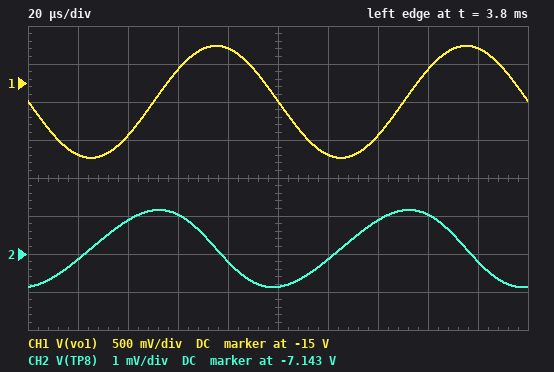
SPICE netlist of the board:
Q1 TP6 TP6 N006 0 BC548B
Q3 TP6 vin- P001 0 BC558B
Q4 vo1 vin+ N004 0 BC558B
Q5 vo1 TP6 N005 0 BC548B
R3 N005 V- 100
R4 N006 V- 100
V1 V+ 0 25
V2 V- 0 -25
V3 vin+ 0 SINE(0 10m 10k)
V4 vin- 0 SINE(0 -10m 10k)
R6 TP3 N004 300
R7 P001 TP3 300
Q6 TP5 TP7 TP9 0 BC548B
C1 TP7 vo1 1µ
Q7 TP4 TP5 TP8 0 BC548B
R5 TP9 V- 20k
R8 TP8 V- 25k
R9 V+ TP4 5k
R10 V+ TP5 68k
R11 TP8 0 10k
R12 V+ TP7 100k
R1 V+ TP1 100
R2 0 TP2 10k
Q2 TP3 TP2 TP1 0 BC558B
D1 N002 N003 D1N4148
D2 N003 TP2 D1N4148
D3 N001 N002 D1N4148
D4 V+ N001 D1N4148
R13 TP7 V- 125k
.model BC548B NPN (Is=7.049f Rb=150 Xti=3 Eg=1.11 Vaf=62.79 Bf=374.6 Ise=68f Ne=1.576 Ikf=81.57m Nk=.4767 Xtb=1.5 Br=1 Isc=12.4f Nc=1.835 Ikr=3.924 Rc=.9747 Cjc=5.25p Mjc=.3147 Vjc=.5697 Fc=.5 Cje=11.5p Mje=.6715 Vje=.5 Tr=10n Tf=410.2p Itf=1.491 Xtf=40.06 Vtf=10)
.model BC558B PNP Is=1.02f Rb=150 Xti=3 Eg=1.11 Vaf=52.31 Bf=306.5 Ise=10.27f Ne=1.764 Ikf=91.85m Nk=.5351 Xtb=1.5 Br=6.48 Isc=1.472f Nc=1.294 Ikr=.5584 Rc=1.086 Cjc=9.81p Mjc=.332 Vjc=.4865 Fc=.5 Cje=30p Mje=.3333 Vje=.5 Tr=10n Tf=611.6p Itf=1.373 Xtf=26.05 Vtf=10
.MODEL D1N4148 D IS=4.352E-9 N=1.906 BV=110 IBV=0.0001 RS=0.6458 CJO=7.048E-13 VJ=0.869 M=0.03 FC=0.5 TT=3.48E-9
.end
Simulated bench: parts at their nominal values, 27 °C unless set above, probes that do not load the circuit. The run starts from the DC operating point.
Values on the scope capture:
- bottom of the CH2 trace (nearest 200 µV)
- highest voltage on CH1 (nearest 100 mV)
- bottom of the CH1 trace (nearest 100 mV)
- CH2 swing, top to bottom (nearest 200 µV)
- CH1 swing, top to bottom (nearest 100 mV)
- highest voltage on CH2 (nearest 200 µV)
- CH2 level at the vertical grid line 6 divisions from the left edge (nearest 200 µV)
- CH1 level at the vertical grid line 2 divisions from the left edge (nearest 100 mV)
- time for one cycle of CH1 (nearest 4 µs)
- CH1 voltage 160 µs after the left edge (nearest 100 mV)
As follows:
-7.1438 V
-14.5 V
-16.0 V
2.0 mV
1.5 V
-7.1418 V
-7.1432 V
-15.7 V
100 µs
-14.8 V
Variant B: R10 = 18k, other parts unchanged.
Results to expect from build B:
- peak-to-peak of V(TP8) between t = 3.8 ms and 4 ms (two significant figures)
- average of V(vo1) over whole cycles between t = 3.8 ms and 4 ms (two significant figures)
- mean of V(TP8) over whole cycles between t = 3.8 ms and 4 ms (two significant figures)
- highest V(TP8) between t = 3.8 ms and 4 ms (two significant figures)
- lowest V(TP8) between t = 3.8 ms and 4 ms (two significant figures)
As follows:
1.9 V
-16 V
1.5 V
2.6 V
760 mV
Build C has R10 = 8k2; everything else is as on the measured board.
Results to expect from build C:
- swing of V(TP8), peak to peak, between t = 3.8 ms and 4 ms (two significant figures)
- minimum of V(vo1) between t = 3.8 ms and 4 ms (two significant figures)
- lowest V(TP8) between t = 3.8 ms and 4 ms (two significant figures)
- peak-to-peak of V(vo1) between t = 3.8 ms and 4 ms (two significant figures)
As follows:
570 mV
-18 V
12 V
5.2 V
